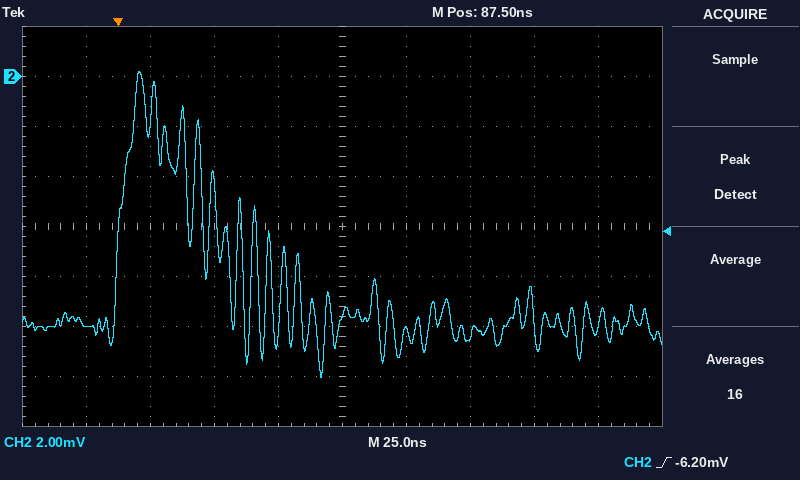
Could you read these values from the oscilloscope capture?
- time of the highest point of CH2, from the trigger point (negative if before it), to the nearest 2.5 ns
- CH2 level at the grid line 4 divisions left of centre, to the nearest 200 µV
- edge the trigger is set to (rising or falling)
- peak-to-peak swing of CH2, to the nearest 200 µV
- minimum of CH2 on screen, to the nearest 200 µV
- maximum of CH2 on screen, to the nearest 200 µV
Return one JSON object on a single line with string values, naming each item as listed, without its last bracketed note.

{"time of the highest point of CH2, from the trigger point (negative if before it), to the nearest 2.5 ns": "+7.5 ns", "CH2 level at the grid line 4 divisions left of centre, to the nearest 200 µV": "-10.0 mV", "edge the trigger is set to": "rising", "peak-to-peak swing of CH2, to the nearest 200 µV": "12.2 mV", "minimum of CH2 on screen, to the nearest 200 µV": "-12.0 mV", "maximum of CH2 on screen, to the nearest 200 µV": "200 µV"}
